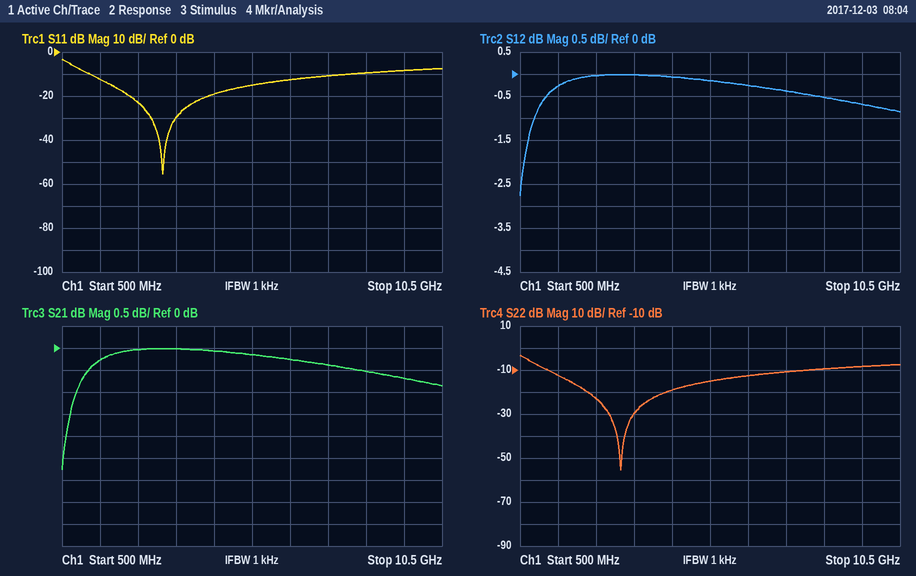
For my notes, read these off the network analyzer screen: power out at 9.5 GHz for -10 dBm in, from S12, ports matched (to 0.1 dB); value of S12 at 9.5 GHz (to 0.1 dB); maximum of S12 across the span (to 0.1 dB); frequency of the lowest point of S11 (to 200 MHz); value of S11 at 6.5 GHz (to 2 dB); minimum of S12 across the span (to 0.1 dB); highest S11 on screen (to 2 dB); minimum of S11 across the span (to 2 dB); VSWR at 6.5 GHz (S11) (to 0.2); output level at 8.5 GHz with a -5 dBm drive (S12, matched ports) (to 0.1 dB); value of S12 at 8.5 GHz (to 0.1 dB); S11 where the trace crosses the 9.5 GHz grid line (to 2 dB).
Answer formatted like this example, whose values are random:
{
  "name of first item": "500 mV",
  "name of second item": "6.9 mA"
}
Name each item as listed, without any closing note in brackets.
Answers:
{
  "power out at 9.5 GHz for -10 dBm in, from S12, ports matched": "-10.7 dBm",
  "value of S12 at 9.5 GHz": "-0.7 dB",
  "maximum of S12 across the span": "0.0 dB",
  "frequency of the lowest point of S11": "3.2 GHz",
  "value of S11 at 6.5 GHz": "-12 dB",
  "minimum of S12 across the span": "-2.8 dB",
  "highest S11 on screen": "-4 dB",
  "minimum of S11 across the span": "-56 dB",
  "VSWR at 6.5 GHz (S11)": "1.6",
  "output level at 8.5 GHz with a -5 dBm drive (S12, matched ports)": "-5.5 dBm",
  "value of S12 at 8.5 GHz": "-0.5 dB",
  "S11 where the trace crosses the 9.5 GHz grid line": "-8 dB"
}
